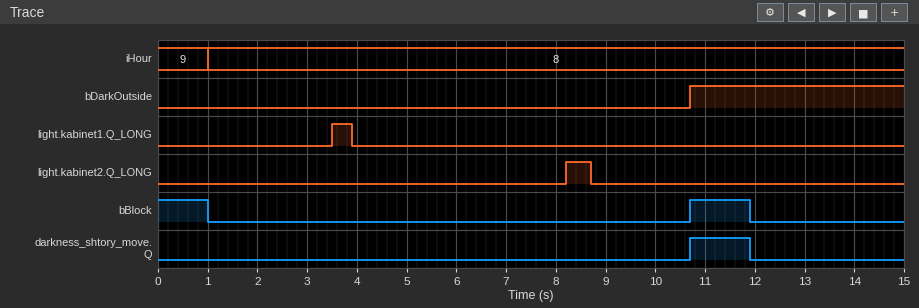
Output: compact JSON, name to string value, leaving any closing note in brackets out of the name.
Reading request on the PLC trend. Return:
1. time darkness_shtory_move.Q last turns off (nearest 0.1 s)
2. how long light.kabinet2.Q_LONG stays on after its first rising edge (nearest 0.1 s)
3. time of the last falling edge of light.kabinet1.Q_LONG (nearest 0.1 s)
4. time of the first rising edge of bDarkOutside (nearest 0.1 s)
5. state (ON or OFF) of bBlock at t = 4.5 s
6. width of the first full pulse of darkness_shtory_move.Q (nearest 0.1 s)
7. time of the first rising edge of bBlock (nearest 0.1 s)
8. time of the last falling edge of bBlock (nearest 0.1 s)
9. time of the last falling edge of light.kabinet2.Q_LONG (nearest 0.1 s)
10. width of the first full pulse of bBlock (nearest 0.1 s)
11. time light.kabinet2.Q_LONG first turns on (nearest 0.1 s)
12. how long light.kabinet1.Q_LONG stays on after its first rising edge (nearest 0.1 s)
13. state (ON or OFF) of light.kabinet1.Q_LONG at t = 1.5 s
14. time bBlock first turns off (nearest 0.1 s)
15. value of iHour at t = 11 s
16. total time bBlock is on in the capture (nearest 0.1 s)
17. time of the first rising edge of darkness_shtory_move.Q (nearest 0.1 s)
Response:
{"time darkness_shtory_move.Q last turns off": "11.9 s", "how long light.kabinet2.Q_LONG stays on after its first rising edge": "0.5 s", "time of the last falling edge of light.kabinet1.Q_LONG": "3.9 s", "time of the first rising edge of bDarkOutside": "10.7 s", "state (ON or OFF) of bBlock at t = 4.5 s": "OFF", "width of the first full pulse of darkness_shtory_move.Q": "1.2 s", "time of the first rising edge of bBlock": "10.7 s", "time of the last falling edge of bBlock": "11.9 s", "time of the last falling edge of light.kabinet2.Q_LONG": "8.7 s", "width of the first full pulse of bBlock": "1.2 s", "time light.kabinet2.Q_LONG first turns on": "8.2 s", "how long light.kabinet1.Q_LONG stays on after its first rising edge": "0.4 s", "state (ON or OFF) of light.kabinet1.Q_LONG at t = 1.5 s": "OFF", "time bBlock first turns off": "1.0 s", "value of iHour at t = 11 s": "8", "total time bBlock is on in the capture": "2.2 s", "time of the first rising edge of darkness_shtory_move.Q": "10.7 s"}
